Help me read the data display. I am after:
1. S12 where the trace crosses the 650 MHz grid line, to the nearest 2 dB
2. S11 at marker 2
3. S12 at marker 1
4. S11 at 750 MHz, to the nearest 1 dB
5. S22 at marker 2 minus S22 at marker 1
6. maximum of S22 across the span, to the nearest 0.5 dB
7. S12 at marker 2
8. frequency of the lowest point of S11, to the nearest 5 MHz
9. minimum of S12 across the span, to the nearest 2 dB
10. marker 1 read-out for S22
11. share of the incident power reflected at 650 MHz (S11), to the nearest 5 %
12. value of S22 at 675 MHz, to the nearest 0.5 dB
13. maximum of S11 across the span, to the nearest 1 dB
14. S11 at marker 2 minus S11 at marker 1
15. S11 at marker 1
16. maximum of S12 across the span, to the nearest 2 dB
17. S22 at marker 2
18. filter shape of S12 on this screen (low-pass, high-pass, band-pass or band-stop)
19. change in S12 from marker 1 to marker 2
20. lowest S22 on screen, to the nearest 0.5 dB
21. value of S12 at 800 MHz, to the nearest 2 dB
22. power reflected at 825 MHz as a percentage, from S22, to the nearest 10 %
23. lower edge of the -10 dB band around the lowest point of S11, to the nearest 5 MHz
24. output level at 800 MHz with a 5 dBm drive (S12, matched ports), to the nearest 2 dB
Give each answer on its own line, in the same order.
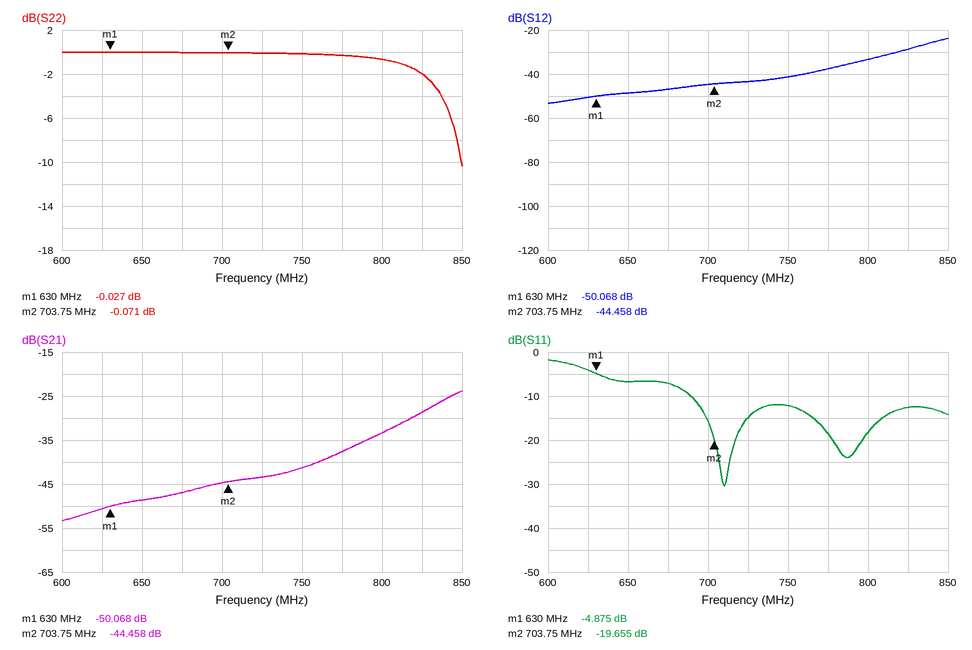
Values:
-48 dB
-19.655 dB
-50.068 dB
-12 dB
-0.044 dB
0.0 dB
-44.458 dB
710 MHz
-54 dB
-0.027 dB
20 %
0.0 dB
-2 dB
-14.780 dB
-4.875 dB
-24 dB
-0.071 dB
high-pass
5.610 dB
-10.5 dB
-34 dB
60 %
690 MHz
-28 dBm
